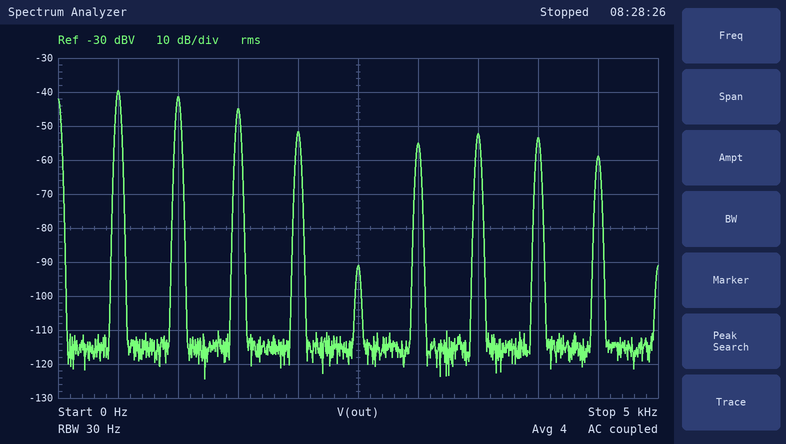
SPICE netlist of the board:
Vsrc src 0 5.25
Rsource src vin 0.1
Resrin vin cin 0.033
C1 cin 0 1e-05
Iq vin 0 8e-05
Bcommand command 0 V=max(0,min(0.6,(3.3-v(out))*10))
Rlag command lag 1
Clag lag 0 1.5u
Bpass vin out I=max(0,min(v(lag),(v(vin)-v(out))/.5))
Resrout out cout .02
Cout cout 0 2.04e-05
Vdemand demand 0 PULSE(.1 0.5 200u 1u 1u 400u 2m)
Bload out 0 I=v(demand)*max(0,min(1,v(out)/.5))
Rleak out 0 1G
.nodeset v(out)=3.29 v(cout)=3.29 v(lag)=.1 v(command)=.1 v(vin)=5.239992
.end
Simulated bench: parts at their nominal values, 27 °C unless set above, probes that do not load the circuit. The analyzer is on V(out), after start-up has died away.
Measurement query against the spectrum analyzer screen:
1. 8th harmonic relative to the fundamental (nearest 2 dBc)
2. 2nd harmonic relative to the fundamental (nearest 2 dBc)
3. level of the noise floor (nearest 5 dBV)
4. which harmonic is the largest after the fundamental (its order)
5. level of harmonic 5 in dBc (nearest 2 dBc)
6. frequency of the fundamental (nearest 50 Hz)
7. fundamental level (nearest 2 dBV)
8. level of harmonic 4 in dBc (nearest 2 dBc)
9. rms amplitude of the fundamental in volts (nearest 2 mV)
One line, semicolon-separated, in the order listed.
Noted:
-14 dBc; -2 dBc; -115 dBV; 2; -52 dBc; 500 Hz; -40 dBV; -12 dBc; 10 mV
